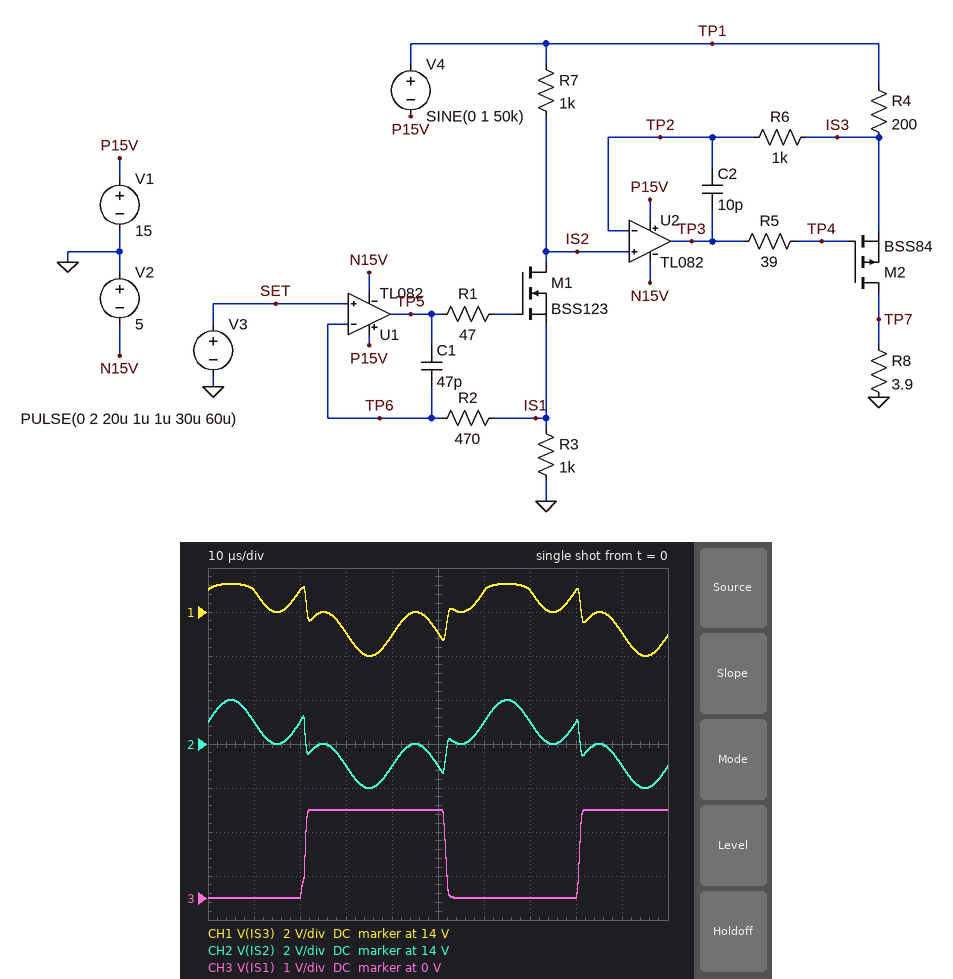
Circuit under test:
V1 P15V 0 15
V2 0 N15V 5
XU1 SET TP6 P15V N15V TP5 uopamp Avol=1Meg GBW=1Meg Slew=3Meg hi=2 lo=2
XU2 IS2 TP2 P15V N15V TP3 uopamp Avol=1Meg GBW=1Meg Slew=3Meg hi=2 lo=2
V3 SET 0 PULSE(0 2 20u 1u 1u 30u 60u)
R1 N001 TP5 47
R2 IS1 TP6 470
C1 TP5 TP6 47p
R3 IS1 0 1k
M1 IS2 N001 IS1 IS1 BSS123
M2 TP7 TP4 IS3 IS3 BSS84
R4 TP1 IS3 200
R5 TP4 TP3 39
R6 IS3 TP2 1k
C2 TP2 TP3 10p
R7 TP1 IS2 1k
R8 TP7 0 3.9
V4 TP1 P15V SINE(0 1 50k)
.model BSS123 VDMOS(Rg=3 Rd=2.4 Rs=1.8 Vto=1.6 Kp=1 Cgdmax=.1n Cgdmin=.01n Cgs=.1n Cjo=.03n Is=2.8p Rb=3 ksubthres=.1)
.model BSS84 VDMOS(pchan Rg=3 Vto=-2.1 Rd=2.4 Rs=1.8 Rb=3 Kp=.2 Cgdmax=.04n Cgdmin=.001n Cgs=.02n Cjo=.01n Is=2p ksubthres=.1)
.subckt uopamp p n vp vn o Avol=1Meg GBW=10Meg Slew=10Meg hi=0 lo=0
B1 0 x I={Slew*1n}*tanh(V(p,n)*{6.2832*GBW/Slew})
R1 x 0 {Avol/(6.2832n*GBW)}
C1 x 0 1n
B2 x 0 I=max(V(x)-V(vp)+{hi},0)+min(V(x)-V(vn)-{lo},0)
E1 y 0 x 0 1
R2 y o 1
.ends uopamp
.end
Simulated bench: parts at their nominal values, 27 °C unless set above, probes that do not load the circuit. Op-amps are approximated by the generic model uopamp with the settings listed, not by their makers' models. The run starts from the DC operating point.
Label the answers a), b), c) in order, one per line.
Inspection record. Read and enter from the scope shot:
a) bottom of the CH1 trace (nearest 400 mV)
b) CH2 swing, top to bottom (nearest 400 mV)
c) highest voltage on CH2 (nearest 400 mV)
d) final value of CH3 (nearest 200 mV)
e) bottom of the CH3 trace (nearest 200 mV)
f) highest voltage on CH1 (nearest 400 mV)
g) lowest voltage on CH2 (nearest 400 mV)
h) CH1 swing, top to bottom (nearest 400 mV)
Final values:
a) 12.0 V
b) 4.0 V
c) 16.0 V
d) 2.0 V
e) 0 V
f) 15.2 V
g) 12.0 V
h) 3.2 V
